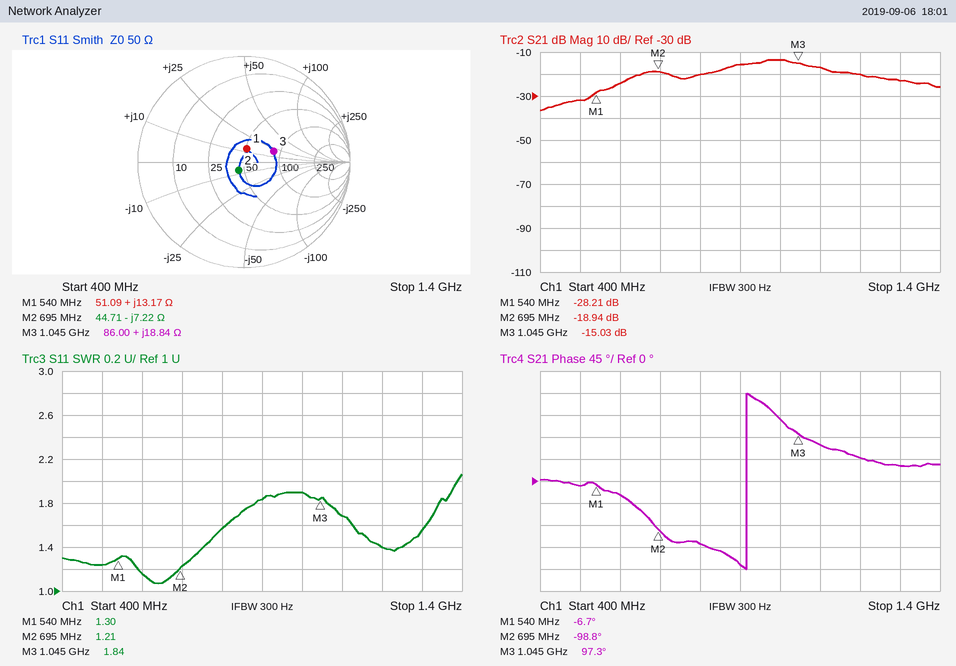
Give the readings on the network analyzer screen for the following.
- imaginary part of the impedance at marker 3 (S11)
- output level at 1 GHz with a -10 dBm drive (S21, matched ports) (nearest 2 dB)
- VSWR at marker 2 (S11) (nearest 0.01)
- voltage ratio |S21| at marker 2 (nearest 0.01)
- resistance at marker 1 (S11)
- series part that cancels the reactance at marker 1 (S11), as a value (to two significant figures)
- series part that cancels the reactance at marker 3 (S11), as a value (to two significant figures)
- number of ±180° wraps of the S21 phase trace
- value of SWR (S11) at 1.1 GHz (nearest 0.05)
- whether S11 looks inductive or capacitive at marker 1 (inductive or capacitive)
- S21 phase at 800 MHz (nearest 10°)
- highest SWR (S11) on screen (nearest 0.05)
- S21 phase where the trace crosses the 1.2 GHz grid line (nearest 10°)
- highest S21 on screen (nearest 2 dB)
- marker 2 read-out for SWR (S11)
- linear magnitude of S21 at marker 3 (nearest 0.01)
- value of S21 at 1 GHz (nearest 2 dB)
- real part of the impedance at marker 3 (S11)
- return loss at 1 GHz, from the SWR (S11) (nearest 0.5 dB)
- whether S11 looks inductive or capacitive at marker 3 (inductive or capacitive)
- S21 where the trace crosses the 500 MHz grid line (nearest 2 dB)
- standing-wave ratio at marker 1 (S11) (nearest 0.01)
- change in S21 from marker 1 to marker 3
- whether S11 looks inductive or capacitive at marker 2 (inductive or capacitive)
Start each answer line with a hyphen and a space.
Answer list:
- +18.84 Ω
- -24 dBm
- 1.21
- 0.11
- 51.09 Ω
- 22 pF
- 8.1 pF
- 1
- 1.70
- inductive
- -130°
- 2.05
- 50°
- -14 dB
- 1.21
- 0.18
- -14 dB
- 86.00 Ω
- 10.0 dB
- inductive
- -32 dB
- 1.30
- 13.18 dB
- capacitive
